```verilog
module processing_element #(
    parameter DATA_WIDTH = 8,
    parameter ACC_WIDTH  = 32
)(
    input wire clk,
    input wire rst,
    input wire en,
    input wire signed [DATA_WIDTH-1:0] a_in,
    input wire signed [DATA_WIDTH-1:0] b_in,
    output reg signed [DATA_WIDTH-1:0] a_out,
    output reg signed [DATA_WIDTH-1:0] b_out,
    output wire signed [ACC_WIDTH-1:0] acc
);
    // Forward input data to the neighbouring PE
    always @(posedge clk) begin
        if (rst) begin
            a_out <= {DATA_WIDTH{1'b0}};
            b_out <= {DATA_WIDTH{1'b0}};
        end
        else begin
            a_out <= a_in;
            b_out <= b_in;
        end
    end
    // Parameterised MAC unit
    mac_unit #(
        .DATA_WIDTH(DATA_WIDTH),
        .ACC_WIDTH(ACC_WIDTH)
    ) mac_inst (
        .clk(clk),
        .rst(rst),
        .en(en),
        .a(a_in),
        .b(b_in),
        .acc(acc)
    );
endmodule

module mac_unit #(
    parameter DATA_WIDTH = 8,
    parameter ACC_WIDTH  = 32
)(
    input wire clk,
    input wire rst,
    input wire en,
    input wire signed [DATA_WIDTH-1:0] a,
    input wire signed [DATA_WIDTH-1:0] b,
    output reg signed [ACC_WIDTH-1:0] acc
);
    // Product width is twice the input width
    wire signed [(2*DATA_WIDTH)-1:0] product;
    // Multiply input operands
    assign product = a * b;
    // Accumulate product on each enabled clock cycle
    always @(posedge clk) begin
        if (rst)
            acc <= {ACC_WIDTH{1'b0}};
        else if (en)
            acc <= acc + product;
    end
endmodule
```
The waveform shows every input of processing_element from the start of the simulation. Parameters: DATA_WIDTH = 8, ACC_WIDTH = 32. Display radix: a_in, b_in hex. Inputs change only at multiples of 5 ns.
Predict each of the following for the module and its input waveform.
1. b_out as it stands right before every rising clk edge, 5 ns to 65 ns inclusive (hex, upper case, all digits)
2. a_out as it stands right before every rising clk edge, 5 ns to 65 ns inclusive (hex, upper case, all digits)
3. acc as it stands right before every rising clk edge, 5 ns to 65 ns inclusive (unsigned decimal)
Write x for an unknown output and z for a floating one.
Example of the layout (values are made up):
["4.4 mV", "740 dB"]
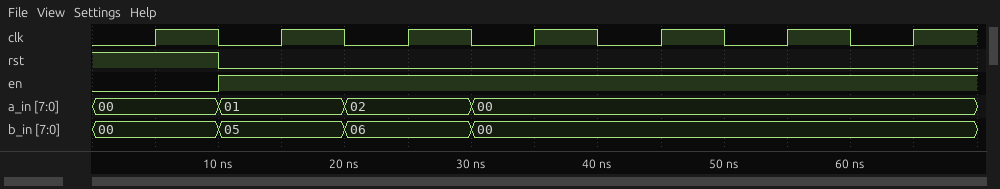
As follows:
["x, 00, 05, 06, 00, 00, 00", "x, 00, 01, 02, 00, 00, 00", "x, 0, 5, 17, 17, 17, 17"]
